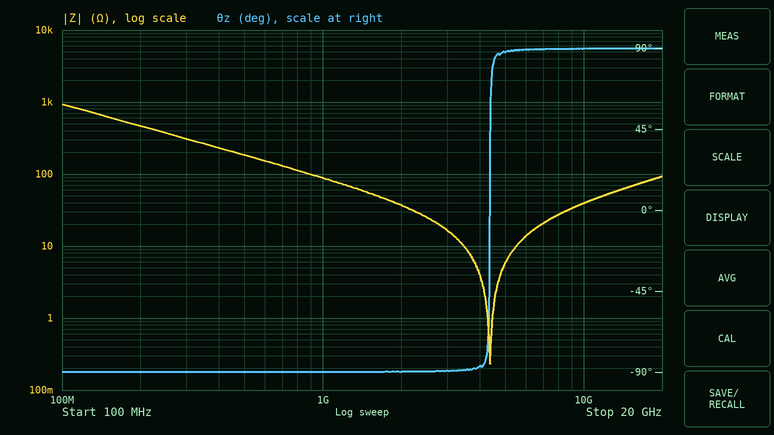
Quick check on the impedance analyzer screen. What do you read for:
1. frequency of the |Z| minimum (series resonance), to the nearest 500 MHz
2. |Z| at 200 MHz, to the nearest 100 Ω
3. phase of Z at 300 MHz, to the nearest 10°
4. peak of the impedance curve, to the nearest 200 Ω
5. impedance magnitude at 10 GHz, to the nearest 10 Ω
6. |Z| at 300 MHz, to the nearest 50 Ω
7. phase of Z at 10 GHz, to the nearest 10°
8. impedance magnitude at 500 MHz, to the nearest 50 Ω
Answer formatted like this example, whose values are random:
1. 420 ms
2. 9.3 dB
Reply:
1. 4.5 GHz
2. 500 Ω
3. -90°
4. 1.0 kΩ
5. 40 Ω
6. 300 Ω
7. 90°
8. 200 Ω
